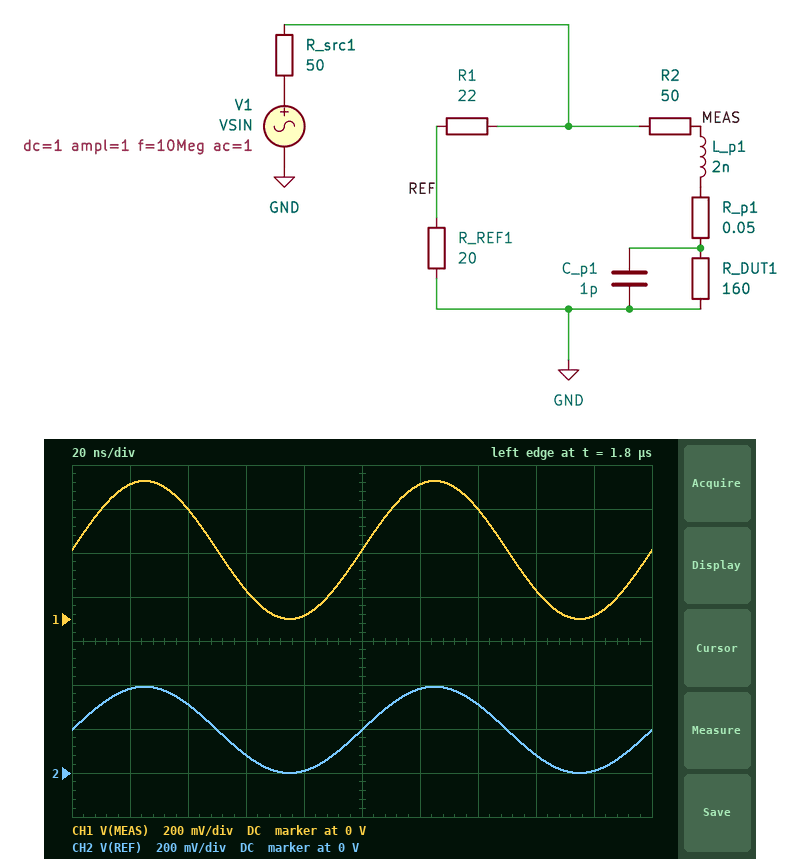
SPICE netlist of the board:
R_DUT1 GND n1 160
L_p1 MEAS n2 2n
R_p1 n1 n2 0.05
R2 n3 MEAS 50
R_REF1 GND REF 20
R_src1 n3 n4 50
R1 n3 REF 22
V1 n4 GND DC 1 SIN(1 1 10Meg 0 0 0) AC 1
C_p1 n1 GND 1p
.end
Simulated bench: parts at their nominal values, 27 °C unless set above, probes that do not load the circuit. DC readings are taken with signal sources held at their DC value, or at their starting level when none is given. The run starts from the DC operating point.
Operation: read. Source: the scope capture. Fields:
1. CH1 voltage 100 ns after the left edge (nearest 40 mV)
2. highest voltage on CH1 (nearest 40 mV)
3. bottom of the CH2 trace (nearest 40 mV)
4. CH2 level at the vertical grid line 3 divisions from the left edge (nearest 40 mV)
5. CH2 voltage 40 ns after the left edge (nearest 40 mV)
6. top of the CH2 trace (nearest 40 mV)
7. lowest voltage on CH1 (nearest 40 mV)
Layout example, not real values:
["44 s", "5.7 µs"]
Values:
["320 mV", "640 mV", "0 V", "80 mV", "320 mV", "400 mV", "0 V"]
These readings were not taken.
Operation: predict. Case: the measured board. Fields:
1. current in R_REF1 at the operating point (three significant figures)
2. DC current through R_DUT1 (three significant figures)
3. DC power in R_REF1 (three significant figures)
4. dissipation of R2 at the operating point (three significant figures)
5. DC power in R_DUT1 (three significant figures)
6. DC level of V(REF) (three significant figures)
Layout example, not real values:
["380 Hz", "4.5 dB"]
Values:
["9.80 mA", "1.96 mA", "1.92 mW", "192 µW", "615 µW", "196 mV"]
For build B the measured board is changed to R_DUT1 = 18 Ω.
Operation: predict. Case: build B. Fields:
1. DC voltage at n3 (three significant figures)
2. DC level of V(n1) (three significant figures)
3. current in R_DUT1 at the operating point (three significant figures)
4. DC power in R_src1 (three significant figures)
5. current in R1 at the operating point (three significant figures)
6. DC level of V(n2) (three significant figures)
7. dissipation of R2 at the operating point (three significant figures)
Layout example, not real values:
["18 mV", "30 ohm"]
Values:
["342 mV", "90.4 mV", "5.02 mA", "8.66 mW", "8.14 mA", "90.7 mV", "1.26 mW"]
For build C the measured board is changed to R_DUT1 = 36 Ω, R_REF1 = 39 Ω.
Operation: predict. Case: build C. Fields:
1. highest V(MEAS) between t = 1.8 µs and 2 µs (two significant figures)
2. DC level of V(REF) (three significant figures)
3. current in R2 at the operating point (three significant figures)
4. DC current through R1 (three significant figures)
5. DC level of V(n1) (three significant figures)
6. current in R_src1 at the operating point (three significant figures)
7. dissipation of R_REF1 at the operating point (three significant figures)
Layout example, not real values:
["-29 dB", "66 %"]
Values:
["350 mV", "266 mV", "4.84 mA", "6.83 mA", "174 mV", "11.7 mA", "1.82 mW"]
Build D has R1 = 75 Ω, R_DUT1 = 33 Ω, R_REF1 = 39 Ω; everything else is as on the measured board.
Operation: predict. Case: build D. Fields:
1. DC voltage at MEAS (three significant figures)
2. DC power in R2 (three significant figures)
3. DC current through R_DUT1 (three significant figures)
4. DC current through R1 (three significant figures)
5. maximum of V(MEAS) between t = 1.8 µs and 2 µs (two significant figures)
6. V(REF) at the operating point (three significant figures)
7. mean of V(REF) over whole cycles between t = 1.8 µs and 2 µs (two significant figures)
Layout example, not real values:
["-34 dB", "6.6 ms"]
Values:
["195 mV", "1.74 mW", "5.90 mA", "4.30 mA", "390 mV", "168 mV", "170 mV"]
